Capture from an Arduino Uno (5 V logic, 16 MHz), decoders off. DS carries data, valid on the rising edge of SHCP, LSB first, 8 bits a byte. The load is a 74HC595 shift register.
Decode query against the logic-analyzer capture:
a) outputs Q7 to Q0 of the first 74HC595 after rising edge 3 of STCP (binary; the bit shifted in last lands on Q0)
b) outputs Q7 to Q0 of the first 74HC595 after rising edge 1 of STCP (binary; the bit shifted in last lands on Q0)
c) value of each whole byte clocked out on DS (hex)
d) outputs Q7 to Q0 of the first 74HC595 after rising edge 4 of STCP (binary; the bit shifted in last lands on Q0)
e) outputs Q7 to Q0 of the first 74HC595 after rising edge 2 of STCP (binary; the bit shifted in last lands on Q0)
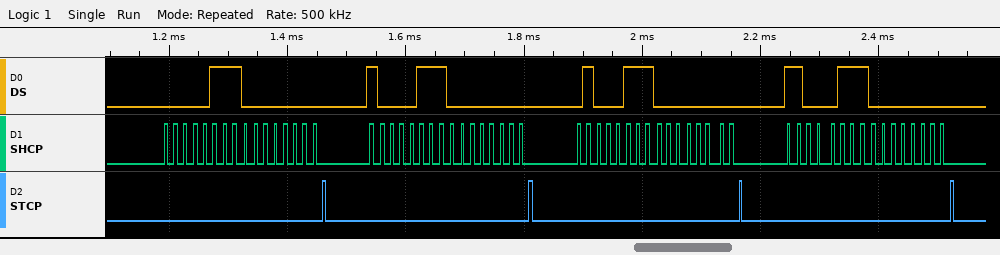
00000000
00000000
E0 00 E1 00 E2 00 E3 00
00000000
00000000
